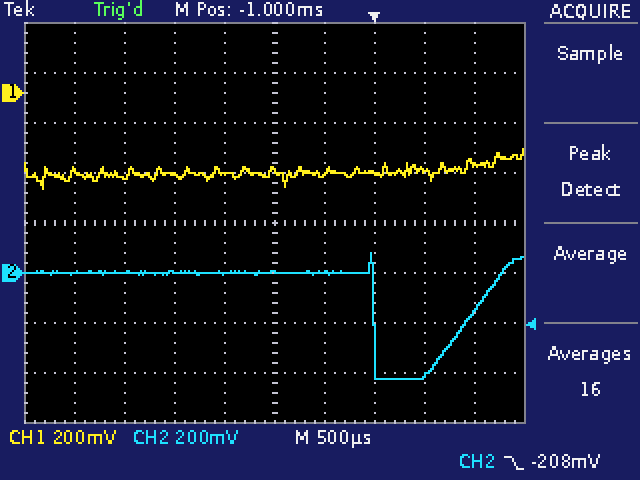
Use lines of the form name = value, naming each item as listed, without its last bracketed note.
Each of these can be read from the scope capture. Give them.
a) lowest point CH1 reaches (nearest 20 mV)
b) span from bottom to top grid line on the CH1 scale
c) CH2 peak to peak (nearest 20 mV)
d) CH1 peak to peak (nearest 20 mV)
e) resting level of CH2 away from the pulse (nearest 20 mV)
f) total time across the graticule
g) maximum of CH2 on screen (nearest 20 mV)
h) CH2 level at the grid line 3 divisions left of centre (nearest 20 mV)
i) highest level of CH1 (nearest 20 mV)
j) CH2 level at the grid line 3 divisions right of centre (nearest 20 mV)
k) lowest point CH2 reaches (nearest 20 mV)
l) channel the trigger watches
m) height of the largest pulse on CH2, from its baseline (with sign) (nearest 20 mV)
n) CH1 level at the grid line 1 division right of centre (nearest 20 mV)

lowest point CH1 reaches = -380 mV
span from bottom to top grid line on the CH1 scale = 1.6 V
CH2 peak to peak = 500 mV
CH1 peak to peak = 160 mV
resting level of CH2 away from the pulse = 0 mV
total time across the graticule = 5 ms
maximum of CH2 on screen = 80 mV
CH2 level at the grid line 3 divisions left of centre = 0 mV
highest level of CH1 = -220 mV
CH2 level at the grid line 3 divisions right of centre = -420 mV
lowest point CH2 reaches = -420 mV
channel the trigger watches = CH2
height of the largest pulse on CH2, from its baseline (with sign) = -420 mV
CH1 level at the grid line 1 division right of centre = -320 mV
